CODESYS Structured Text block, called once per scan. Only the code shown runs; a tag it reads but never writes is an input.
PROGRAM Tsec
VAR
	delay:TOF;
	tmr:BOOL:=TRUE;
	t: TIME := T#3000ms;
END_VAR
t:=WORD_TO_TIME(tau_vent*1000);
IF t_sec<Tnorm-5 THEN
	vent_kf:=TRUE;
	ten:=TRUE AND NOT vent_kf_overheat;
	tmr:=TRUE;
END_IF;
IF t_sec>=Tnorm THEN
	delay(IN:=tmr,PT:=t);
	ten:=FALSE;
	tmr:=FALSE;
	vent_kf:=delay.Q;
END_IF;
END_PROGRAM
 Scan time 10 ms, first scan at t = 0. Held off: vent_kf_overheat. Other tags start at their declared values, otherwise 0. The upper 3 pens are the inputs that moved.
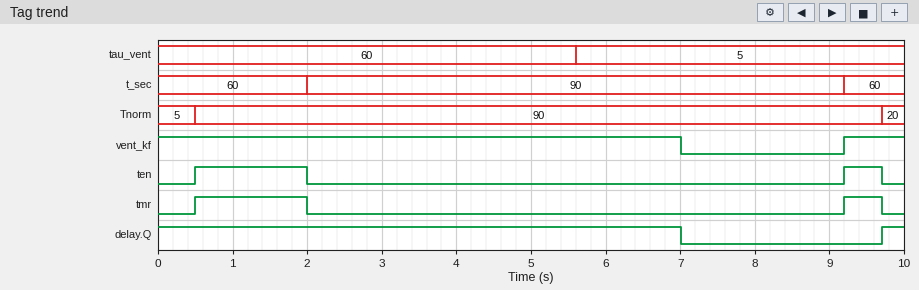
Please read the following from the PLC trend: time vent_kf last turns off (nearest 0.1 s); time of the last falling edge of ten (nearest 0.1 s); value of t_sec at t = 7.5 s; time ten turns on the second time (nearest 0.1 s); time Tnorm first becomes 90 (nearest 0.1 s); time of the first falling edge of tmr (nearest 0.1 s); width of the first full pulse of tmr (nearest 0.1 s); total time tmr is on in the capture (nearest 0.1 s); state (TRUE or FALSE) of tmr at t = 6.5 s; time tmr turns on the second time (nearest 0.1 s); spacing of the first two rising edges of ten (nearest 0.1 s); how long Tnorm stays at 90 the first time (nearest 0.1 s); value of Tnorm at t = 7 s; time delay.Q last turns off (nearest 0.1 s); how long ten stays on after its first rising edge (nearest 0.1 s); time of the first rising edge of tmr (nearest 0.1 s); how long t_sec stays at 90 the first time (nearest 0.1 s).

7.0 s
9.7 s
90
9.2 s
0.5 s
2.0 s
1.5 s
2.0 s
FALSE
9.2 s
8.7 s
9.2 s
90
7.0 s
1.5 s
0.5 s
7.2 s
